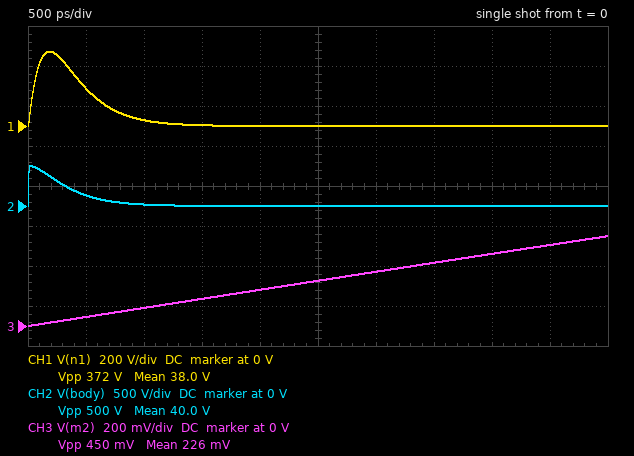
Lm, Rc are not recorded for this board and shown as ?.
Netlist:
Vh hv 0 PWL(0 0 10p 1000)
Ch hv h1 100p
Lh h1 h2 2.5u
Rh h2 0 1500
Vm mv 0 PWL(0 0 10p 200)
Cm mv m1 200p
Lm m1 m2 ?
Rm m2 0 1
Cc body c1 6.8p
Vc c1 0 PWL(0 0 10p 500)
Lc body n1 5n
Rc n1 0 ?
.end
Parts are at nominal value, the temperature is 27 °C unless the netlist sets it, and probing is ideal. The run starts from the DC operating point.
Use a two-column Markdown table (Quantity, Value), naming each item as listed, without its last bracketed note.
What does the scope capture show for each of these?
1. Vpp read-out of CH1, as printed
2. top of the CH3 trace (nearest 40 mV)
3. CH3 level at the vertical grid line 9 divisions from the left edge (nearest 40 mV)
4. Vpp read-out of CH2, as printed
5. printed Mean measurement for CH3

| Quantity | Value |
|---|---|
| Vpp read-out of CH1, as printed | 372 V |
| top of the CH3 trace | 440 mV |
| CH3 level at the vertical grid line 9 divisions from the left edge | 400 mV |
| Vpp read-out of CH2, as printed | 500 V |
| printed Mean measurement for CH3 | 226 mV |
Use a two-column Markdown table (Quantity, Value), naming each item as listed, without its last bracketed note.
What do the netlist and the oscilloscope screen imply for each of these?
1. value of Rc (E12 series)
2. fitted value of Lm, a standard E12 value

| Quantity | Value |
|---|---|
| value of Rc | 56 Ω |
| fitted value of Lm, a standard E12 value | 2.2 µH |
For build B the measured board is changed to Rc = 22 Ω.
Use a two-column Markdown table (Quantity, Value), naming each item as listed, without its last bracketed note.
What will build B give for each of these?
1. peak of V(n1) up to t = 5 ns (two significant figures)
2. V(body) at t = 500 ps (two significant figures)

| Quantity | Value |
|---|---|
| peak of V(n1) up to t = 5 ns | 240 V |
| V(body) at t = 500 ps | -83 V |
